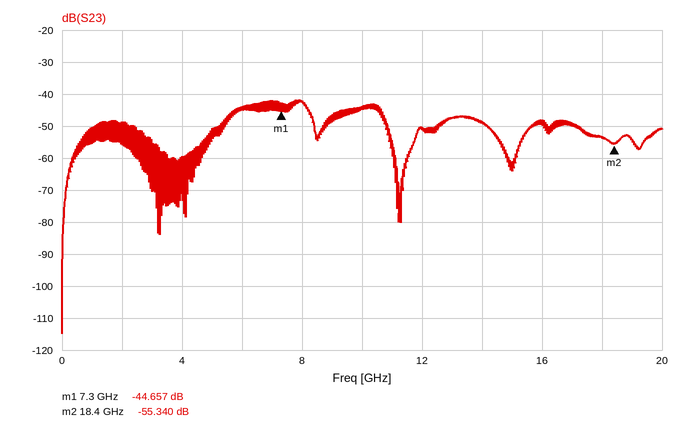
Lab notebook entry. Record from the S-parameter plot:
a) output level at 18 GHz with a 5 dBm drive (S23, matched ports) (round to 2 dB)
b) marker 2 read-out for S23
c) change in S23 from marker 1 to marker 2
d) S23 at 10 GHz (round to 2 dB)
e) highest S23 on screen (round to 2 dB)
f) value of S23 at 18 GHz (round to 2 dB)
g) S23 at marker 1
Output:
-48 dBm
-55.340 dB
-10.683 dB
-44 dB
-42 dB
-54 dB
-44.657 dB
